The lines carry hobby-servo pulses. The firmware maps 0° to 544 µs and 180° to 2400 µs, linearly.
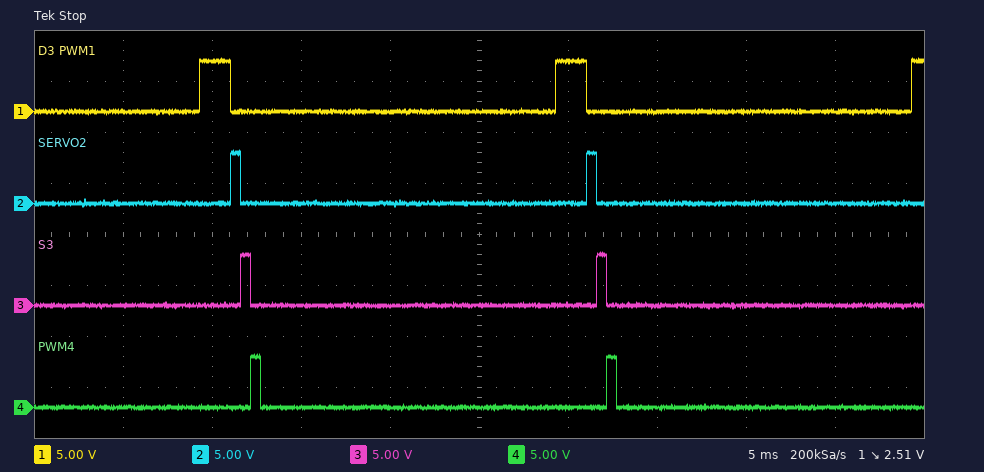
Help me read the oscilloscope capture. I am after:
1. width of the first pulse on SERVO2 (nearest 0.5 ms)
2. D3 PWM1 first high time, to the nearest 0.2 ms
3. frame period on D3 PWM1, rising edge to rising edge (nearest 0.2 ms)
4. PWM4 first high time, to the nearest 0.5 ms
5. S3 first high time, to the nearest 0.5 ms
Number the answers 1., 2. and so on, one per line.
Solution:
1. 0.5 ms
2. 1.8 ms
3. 20.0 ms
4. 0.5 ms
5. 0.5 ms
